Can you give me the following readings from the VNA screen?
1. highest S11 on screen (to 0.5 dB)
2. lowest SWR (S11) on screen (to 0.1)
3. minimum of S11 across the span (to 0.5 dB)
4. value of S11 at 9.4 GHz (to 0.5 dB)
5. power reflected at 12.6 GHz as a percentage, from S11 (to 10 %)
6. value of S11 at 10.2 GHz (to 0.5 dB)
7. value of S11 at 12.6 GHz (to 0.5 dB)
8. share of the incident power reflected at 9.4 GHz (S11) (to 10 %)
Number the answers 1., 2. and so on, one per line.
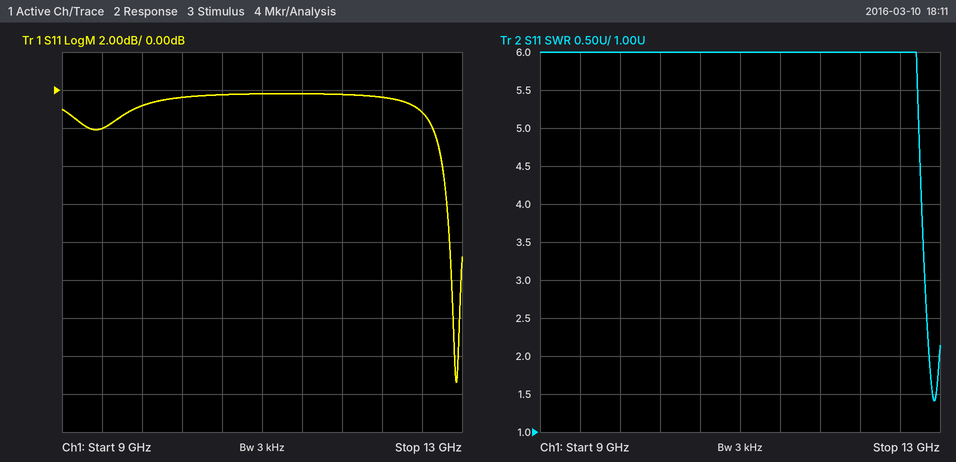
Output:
1. 0.0 dB
2. 1.4
3. -15.5 dB
4. -2.0 dB
5. 80 %
6. -0.5 dB
7. -1.0 dB
8. 60 %
